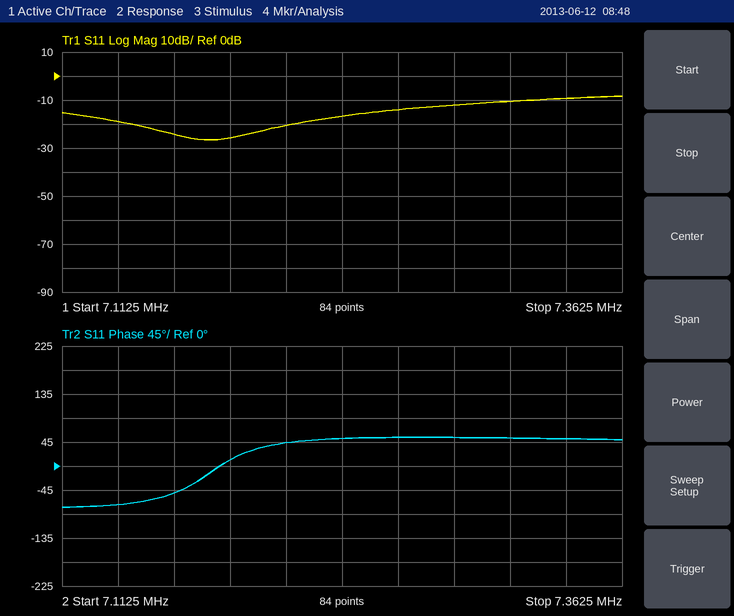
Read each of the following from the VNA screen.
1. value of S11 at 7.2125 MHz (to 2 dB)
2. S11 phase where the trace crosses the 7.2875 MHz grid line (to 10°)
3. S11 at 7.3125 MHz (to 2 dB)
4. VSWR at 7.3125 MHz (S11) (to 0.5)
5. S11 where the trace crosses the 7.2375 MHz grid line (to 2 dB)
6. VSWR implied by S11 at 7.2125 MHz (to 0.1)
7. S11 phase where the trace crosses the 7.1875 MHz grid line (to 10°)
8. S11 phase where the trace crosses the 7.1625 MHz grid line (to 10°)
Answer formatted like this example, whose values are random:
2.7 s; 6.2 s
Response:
-20 dB; 50°; -10 dB; 2.0; -16 dB; 1.2; 10°; -50°
